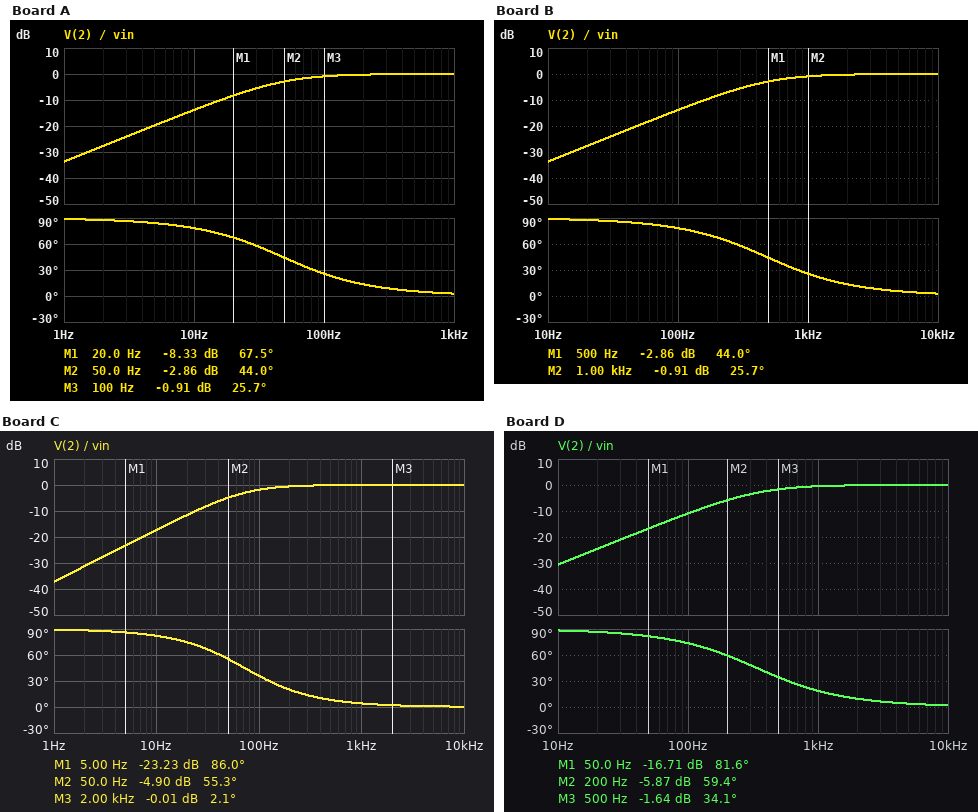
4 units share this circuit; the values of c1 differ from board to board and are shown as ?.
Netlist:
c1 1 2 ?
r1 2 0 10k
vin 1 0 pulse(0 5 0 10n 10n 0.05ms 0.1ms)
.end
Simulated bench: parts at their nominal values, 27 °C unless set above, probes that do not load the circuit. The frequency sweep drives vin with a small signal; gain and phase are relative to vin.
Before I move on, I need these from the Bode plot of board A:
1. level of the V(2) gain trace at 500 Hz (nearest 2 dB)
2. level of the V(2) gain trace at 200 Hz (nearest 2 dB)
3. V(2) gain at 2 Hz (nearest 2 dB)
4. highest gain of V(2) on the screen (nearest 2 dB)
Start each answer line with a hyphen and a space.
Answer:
- 0 dB
- 0 dB
- -28 dB
- 0 dB
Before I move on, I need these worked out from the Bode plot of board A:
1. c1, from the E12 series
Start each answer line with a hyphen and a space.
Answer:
- 330 nF
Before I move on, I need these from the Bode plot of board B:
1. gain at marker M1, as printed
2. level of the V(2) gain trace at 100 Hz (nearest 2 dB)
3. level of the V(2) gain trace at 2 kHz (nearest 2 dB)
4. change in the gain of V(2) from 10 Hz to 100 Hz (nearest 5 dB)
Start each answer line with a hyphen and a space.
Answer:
- -2.86 dB
- -14 dB
- 0 dB
- 20 dB
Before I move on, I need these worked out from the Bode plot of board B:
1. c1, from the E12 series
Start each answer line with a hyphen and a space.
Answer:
- 33 nF
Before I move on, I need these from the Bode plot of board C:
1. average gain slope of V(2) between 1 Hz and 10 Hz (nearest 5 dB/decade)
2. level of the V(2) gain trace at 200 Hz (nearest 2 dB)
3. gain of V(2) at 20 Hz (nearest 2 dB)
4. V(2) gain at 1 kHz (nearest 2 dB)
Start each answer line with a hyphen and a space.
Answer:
- 20 dB/decade
- 0 dB
- -12 dB
- 0 dB
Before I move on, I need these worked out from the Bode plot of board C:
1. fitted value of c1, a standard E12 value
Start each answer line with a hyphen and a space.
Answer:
- 220 nF
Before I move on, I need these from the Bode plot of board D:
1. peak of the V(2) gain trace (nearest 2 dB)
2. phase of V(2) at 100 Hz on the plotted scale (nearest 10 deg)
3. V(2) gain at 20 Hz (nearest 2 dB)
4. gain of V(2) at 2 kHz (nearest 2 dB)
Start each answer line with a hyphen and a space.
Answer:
- 0 dB
- 70 deg
- -24 dB
- 0 dB
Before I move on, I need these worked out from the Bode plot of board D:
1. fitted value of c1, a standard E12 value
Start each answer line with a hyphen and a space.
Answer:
- 47 nF
